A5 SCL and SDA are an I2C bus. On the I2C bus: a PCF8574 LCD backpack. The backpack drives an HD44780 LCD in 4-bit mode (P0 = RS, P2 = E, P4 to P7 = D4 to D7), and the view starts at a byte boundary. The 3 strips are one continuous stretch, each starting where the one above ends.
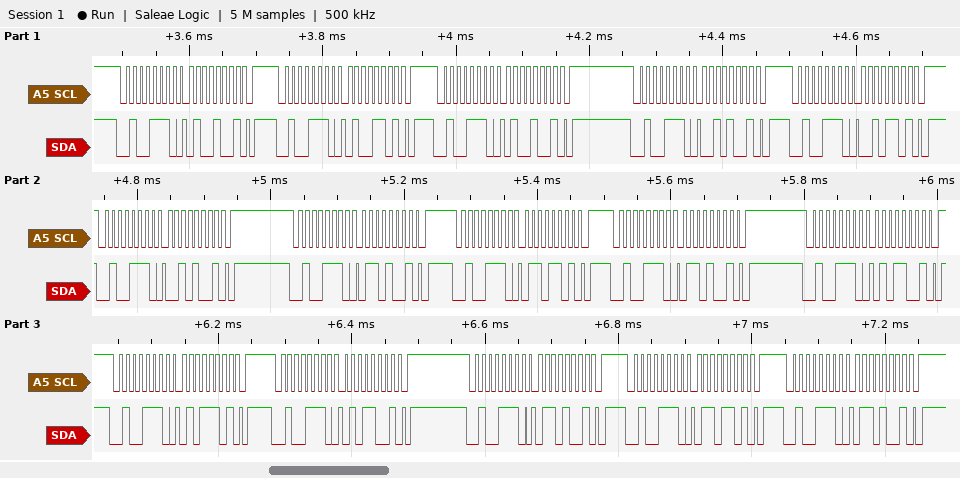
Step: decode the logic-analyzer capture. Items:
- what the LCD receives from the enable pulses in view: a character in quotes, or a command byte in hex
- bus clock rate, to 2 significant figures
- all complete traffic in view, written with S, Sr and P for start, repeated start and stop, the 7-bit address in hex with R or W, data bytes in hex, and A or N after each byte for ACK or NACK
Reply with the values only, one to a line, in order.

'B' 'e'
100 kHz
S 27W A 49 A P S 27W A 4D A P S 27W A 49 A P S 27W A 29 A P S 27W A 2D A P S 27W A 29 A P S 27W A 69 A P S 27W A 6D A P S 27W A 69 A P S 27W A 59 A P S 27W A 5D A P S 27W A 59 A P S 27W A 69 A P S 27W A 6D A P S 27W A 69 A P
